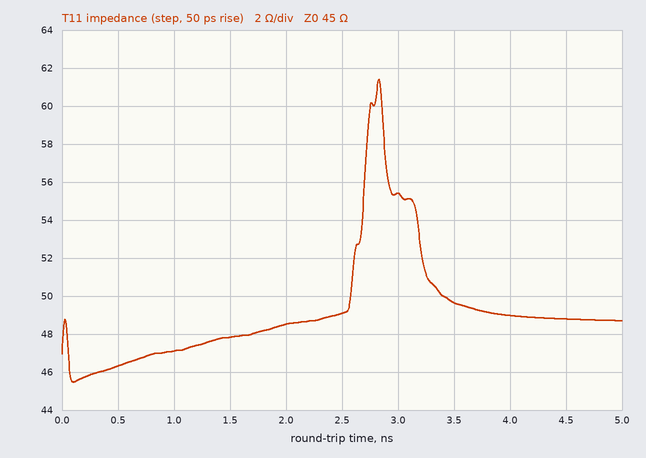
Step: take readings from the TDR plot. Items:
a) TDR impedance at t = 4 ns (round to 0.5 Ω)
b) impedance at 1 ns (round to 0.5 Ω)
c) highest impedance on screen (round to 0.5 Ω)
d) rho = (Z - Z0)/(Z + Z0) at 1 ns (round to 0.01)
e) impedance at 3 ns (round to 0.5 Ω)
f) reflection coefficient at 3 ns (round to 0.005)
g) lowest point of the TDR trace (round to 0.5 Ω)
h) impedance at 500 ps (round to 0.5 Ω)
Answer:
49.0 Ω
47.0 Ω
61.5 Ω
+0.02
55.5 Ω
+0.105
45.5 Ω
46.5 Ω
